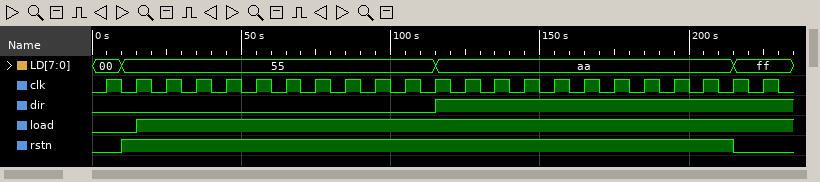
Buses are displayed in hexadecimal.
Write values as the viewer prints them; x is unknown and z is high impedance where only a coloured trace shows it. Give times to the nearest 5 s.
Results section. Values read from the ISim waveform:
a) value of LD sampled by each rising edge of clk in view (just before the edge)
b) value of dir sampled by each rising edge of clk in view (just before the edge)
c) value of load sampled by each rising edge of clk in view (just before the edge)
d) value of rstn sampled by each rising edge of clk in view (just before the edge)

00, 55, 55, 55, 55, 55, 55, 55, 55, 55, 55, 55, aa, aa, aa, aa, aa, aa, aa, aa, aa, aa, ff
0 0 0 0 0 0 0 0 0 0 0 0 1 1 1 1 1 1 1 1 1 1 1
0 0 1 1 1 1 1 1 1 1 1 1 1 1 1 1 1 1 1 1 1 1 1
0 1 1 1 1 1 1 1 1 1 1 1 1 1 1 1 1 1 1 1 1 1 0
